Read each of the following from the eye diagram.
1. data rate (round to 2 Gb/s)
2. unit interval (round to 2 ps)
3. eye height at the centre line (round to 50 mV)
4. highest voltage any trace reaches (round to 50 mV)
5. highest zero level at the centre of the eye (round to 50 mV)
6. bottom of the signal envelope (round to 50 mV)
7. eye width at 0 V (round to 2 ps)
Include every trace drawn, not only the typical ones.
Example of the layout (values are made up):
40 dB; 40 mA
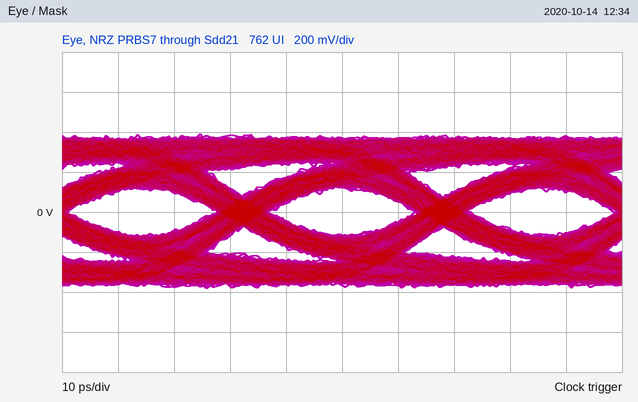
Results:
28 Gb/s; 36 ps; 250 mV; 400 mV; -100 mV; -400 mV; 26 ps
